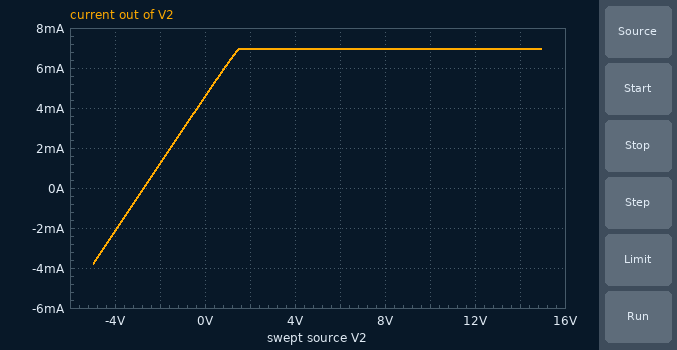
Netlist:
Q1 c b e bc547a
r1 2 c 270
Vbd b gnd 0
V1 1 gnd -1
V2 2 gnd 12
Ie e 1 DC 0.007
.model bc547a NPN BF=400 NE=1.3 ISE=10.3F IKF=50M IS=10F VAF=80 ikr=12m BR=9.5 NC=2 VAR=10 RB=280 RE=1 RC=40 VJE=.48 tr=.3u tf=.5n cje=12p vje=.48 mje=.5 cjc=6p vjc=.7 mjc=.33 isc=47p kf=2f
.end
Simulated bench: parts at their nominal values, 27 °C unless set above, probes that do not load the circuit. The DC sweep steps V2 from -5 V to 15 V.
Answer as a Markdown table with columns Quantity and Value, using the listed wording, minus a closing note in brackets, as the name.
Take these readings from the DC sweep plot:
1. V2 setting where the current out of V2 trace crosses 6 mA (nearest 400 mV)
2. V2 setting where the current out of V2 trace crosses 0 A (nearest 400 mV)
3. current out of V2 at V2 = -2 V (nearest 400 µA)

| Quantity | Value |
|---|---|
| V2 setting where the current out of V2 trace crosses 6 mA | 800 mV |
| V2 setting where the current out of V2 trace crosses 0 A | -2.8 V |
| current out of V2 at V2 = -2 V | 1.2 mA |
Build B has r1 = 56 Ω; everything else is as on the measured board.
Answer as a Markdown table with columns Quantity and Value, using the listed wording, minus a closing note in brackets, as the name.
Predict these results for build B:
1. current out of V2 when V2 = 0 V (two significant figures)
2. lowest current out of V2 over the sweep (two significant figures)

| Quantity | Value |
|---|---|
| current out of V2 when V2 = 0 V | 6.9 mA |
| lowest current out of V2 over the sweep | -6.0 mA |
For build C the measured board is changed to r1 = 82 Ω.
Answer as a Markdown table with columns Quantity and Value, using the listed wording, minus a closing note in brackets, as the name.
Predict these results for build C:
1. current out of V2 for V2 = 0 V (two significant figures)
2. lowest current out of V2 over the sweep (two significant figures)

| Quantity | Value |
|---|---|
| current out of V2 for V2 = 0 V | 6.6 mA |
| lowest current out of V2 over the sweep | -5.6 mA |
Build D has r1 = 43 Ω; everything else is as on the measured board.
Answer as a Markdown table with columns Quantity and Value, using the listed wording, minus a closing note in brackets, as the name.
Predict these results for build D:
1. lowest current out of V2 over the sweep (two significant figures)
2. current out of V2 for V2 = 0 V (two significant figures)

| Quantity | Value |
|---|---|
| lowest current out of V2 over the sweep | -6.2 mA |
| current out of V2 for V2 = 0 V | 7.0 mA |
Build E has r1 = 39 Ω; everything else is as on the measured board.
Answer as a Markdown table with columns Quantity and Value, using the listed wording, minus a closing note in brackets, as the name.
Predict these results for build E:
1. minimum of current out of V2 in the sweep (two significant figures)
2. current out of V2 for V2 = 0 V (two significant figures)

| Quantity | Value |
|---|---|
| minimum of current out of V2 in the sweep | -6.3 mA |
| current out of V2 for V2 = 0 V | 7.0 mA |
